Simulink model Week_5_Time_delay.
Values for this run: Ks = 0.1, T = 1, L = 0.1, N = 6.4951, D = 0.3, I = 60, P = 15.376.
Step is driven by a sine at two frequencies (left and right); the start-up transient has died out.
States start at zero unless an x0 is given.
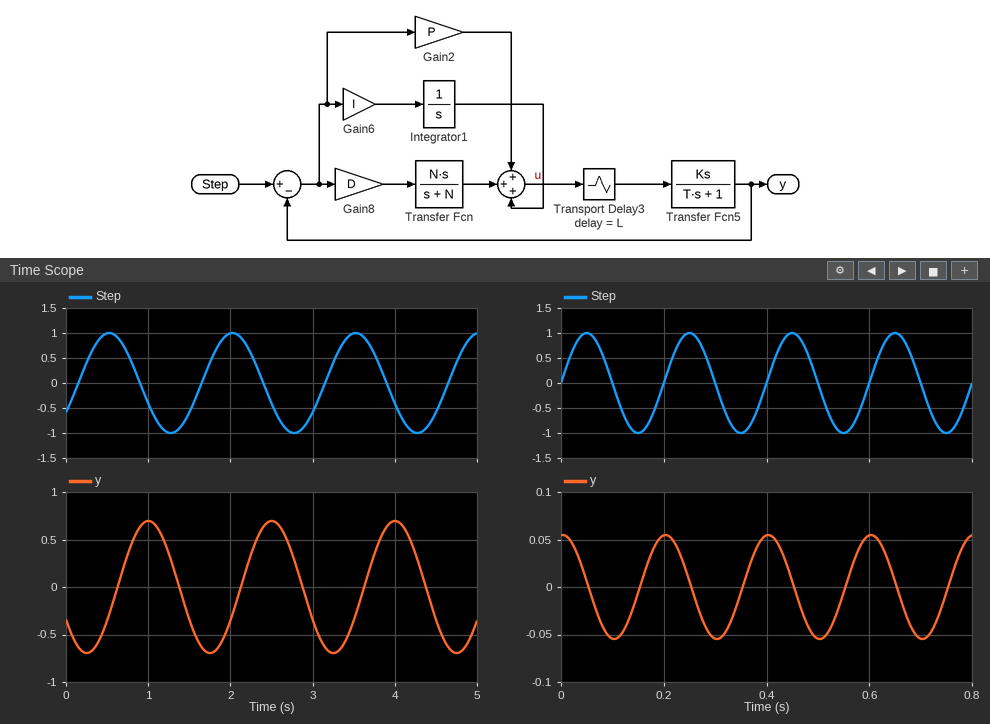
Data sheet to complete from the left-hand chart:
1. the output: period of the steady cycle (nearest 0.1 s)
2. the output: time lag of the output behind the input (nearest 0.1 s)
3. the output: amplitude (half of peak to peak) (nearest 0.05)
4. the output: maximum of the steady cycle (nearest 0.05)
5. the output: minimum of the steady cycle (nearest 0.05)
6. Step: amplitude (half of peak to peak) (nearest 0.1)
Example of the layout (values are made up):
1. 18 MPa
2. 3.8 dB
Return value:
1. 1.5 s
2. 0.5 s
3. 0.70
4. 0.70
5. -0.70
6. 1.0
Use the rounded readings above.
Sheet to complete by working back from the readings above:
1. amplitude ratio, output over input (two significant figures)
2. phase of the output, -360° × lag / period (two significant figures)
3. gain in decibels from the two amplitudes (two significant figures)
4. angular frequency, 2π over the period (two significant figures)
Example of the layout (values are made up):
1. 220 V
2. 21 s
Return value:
1. 0.70
2. -120°
3. -3.1 dB
4. 4.2 rad/s
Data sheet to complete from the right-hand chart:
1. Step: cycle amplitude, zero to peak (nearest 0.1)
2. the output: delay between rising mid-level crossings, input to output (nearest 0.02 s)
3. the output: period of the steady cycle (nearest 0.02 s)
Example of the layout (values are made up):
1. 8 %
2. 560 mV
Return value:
1. 1.0
2. 0.16 s
3. 0.20 s
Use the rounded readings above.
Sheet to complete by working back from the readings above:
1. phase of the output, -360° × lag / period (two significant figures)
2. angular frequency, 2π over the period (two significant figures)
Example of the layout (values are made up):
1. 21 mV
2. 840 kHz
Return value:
1. -290°
2. 31 rad/s
